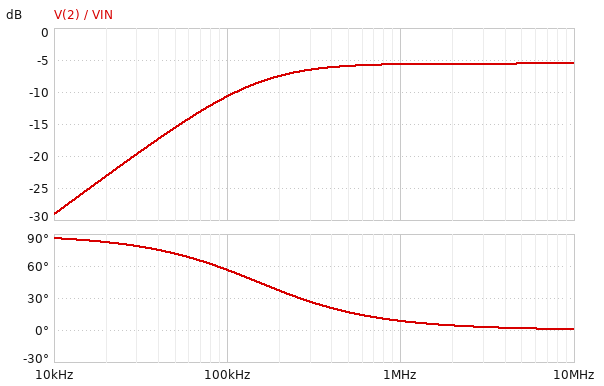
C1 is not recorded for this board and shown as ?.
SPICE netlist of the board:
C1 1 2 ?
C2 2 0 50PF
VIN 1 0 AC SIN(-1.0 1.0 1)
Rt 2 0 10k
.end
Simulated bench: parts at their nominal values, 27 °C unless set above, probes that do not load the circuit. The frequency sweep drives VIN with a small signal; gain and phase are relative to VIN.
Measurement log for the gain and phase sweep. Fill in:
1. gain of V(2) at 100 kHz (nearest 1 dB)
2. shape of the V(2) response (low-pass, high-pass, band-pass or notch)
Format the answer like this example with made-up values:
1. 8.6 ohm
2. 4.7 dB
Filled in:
1. -11 dB
2. high-pass
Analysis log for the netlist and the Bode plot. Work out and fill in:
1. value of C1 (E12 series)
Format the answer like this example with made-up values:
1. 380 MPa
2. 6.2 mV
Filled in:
1. 56 pF
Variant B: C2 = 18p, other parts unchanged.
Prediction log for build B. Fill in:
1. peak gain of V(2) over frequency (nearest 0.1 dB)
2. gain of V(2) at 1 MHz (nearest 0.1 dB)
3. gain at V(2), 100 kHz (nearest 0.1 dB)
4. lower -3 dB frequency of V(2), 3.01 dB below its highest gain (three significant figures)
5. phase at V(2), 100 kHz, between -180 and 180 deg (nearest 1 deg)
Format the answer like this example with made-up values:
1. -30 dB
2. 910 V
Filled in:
1. -2.4 dB
2. -2.6 dB
3. -9.9 dB
4. 215 kHz
5. 65 deg
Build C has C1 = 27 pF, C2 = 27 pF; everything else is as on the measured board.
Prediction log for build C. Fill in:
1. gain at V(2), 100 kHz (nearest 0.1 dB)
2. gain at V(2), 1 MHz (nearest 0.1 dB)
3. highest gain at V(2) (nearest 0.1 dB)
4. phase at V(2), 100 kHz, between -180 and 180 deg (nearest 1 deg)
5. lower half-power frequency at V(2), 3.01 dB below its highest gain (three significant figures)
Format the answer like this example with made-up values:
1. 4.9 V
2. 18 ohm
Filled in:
1. -15.9 dB
2. -6.4 dB
3. -6.0 dB
4. 71 deg
5. 295 kHz
